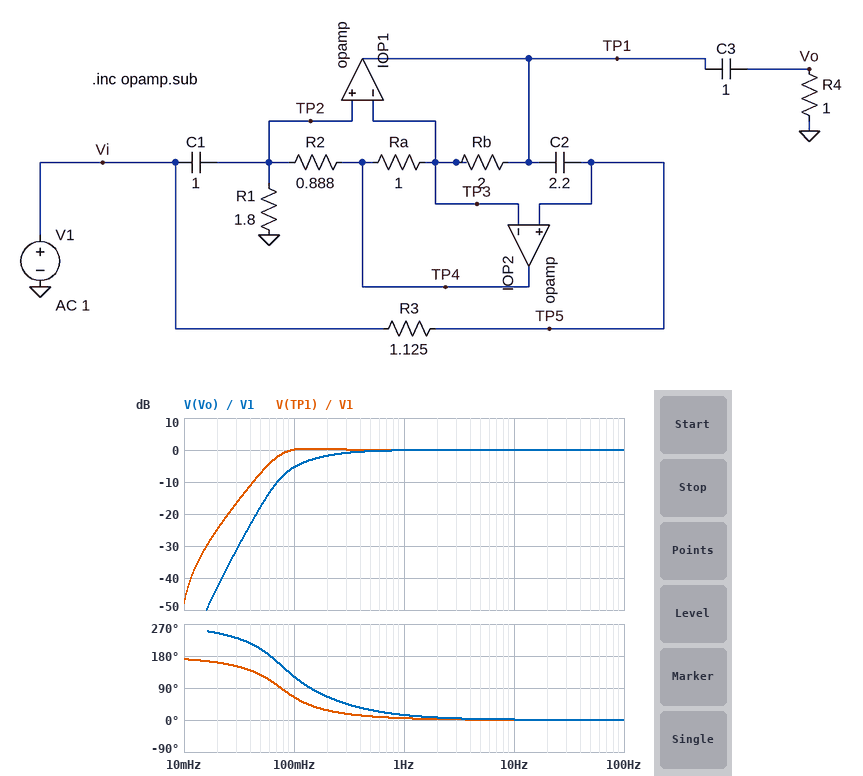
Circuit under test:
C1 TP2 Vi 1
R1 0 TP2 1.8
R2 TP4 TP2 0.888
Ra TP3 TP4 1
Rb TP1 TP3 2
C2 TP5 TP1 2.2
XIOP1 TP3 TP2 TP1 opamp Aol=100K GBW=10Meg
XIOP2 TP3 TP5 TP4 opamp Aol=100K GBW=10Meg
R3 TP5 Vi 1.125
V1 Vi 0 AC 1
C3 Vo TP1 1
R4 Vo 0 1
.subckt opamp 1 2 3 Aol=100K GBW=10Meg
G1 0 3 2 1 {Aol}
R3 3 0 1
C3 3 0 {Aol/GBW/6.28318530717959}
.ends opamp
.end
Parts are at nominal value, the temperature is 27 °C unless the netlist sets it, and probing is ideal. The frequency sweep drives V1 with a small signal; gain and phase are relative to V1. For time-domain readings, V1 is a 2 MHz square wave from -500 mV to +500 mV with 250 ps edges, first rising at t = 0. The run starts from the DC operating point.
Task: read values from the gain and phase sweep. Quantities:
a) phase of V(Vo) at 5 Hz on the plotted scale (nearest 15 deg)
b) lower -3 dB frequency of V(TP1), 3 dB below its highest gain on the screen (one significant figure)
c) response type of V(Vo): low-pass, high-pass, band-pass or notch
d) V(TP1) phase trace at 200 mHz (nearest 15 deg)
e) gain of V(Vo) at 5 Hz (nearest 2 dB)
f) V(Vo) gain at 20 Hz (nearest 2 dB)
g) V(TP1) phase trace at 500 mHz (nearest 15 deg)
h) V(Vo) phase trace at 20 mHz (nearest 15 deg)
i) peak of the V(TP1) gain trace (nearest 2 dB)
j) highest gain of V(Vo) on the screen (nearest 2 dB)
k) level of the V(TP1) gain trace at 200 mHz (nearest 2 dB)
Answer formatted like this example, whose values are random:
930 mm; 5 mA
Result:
0 deg; 70 mHz; high-pass; 30 deg; 0 dB; 0 dB; 15 deg; 240 deg; 0 dB; 0 dB; 0 dB
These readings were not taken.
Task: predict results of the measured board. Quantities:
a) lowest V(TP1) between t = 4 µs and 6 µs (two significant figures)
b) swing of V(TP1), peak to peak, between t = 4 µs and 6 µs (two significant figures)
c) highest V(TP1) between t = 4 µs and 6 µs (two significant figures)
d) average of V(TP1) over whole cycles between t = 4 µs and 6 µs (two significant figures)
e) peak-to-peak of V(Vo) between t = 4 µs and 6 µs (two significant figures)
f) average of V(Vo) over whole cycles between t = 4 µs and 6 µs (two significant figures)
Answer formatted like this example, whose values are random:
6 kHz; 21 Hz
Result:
-250 mV; 1.5 V; 1.2 V; 490 mV; 1.5 V; 500 mV
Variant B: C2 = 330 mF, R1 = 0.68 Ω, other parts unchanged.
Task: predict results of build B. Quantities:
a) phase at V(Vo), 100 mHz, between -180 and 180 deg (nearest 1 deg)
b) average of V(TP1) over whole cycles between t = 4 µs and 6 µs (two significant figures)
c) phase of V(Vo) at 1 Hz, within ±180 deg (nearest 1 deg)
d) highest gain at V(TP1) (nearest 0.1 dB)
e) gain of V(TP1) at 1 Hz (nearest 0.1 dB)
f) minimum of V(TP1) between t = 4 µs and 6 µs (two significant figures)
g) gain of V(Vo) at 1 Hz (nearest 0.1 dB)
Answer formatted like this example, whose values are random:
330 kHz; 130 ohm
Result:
-162 deg; 1.3 V; 23 deg; 6.9 dB; 0.6 dB; 560 mV; 0.5 dB
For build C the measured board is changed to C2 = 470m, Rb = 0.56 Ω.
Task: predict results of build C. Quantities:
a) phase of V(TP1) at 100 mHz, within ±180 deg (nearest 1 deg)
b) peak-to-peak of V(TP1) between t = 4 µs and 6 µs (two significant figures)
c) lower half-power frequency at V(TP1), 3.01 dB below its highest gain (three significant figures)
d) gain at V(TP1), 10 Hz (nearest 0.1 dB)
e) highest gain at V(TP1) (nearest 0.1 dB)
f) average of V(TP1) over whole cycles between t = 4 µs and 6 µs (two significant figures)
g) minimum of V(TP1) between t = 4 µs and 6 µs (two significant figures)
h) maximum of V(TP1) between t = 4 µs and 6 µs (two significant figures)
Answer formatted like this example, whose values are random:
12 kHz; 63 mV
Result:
-6 deg; 1.3 V; 308 mHz; 0 dB; 2.3 dB; 140 mV; -530 mV; 810 mV
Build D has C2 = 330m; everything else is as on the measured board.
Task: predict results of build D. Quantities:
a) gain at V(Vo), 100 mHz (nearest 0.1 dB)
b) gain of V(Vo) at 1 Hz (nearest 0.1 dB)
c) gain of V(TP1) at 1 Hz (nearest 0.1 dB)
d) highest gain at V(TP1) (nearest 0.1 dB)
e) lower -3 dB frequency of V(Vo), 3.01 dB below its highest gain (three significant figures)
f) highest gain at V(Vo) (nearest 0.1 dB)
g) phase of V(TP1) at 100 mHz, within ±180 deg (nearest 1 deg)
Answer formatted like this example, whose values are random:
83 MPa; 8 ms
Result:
-15.4 dB; 0.2 dB; 0.3 dB; 7.0 dB; 174 mHz; 5.1 dB; 163 deg
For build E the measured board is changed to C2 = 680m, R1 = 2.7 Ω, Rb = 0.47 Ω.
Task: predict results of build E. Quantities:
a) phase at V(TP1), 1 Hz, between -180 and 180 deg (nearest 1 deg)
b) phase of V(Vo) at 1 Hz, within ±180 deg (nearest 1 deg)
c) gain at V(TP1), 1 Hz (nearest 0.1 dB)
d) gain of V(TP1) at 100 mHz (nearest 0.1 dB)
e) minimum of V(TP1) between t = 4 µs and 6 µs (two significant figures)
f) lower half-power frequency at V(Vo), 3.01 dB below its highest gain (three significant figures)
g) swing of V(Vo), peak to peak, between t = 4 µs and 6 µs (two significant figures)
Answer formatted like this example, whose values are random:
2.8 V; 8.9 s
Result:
4 deg; 13 deg; 0.1 dB; -1.7 dB; -580 mV; 286 mHz; 1.3 V
